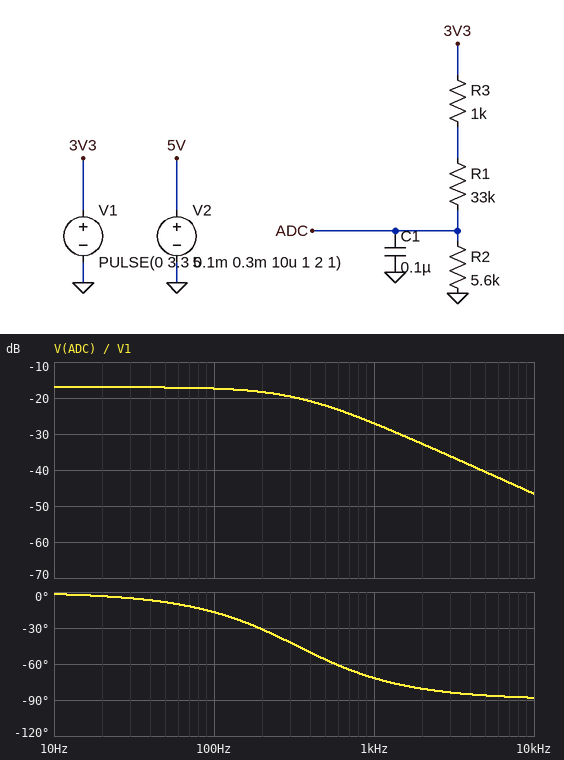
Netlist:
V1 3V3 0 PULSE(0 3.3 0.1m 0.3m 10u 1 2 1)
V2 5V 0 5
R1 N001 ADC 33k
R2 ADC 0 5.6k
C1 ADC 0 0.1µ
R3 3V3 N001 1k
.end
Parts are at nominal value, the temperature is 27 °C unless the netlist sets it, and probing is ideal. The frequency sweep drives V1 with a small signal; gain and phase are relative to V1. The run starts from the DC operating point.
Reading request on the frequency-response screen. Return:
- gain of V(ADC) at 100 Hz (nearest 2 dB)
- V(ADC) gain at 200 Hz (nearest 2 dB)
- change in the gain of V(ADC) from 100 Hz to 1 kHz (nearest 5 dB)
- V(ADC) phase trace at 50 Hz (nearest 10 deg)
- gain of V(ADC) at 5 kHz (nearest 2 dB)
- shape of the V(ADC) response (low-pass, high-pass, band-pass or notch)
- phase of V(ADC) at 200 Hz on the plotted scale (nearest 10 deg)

-18 dB
-18 dB
-10 dB
-10 deg
-40 dB
low-pass
-30 deg
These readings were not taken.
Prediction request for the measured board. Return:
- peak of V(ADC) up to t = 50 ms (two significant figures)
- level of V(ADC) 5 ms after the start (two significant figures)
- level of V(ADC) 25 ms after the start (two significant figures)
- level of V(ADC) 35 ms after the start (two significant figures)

470 mV
470 mV
470 mV
470 mV
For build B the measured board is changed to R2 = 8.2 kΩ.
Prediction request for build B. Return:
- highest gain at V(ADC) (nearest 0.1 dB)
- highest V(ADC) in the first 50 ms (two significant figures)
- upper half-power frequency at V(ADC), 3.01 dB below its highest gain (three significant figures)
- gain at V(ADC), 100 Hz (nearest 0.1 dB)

-14.2 dB
640 mV
241 Hz
-14.9 dB
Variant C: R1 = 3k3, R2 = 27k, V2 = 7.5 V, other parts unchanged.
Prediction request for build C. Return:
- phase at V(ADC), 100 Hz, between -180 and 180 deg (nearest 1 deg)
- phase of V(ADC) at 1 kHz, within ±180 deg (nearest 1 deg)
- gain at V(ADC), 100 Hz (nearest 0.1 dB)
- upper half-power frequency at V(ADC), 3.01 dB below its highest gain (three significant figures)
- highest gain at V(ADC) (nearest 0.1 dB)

-13 deg
-67 deg
-1.5 dB
429 Hz
-1.3 dB
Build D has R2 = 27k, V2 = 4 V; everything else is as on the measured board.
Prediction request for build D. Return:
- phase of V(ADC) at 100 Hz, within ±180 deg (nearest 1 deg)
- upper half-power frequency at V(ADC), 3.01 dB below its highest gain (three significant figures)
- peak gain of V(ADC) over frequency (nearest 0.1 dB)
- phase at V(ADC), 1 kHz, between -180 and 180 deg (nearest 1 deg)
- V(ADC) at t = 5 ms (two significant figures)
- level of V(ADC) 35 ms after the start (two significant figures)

-43 deg
106 Hz
-7.1 dB
-84 deg
1.4 V
1.5 V
